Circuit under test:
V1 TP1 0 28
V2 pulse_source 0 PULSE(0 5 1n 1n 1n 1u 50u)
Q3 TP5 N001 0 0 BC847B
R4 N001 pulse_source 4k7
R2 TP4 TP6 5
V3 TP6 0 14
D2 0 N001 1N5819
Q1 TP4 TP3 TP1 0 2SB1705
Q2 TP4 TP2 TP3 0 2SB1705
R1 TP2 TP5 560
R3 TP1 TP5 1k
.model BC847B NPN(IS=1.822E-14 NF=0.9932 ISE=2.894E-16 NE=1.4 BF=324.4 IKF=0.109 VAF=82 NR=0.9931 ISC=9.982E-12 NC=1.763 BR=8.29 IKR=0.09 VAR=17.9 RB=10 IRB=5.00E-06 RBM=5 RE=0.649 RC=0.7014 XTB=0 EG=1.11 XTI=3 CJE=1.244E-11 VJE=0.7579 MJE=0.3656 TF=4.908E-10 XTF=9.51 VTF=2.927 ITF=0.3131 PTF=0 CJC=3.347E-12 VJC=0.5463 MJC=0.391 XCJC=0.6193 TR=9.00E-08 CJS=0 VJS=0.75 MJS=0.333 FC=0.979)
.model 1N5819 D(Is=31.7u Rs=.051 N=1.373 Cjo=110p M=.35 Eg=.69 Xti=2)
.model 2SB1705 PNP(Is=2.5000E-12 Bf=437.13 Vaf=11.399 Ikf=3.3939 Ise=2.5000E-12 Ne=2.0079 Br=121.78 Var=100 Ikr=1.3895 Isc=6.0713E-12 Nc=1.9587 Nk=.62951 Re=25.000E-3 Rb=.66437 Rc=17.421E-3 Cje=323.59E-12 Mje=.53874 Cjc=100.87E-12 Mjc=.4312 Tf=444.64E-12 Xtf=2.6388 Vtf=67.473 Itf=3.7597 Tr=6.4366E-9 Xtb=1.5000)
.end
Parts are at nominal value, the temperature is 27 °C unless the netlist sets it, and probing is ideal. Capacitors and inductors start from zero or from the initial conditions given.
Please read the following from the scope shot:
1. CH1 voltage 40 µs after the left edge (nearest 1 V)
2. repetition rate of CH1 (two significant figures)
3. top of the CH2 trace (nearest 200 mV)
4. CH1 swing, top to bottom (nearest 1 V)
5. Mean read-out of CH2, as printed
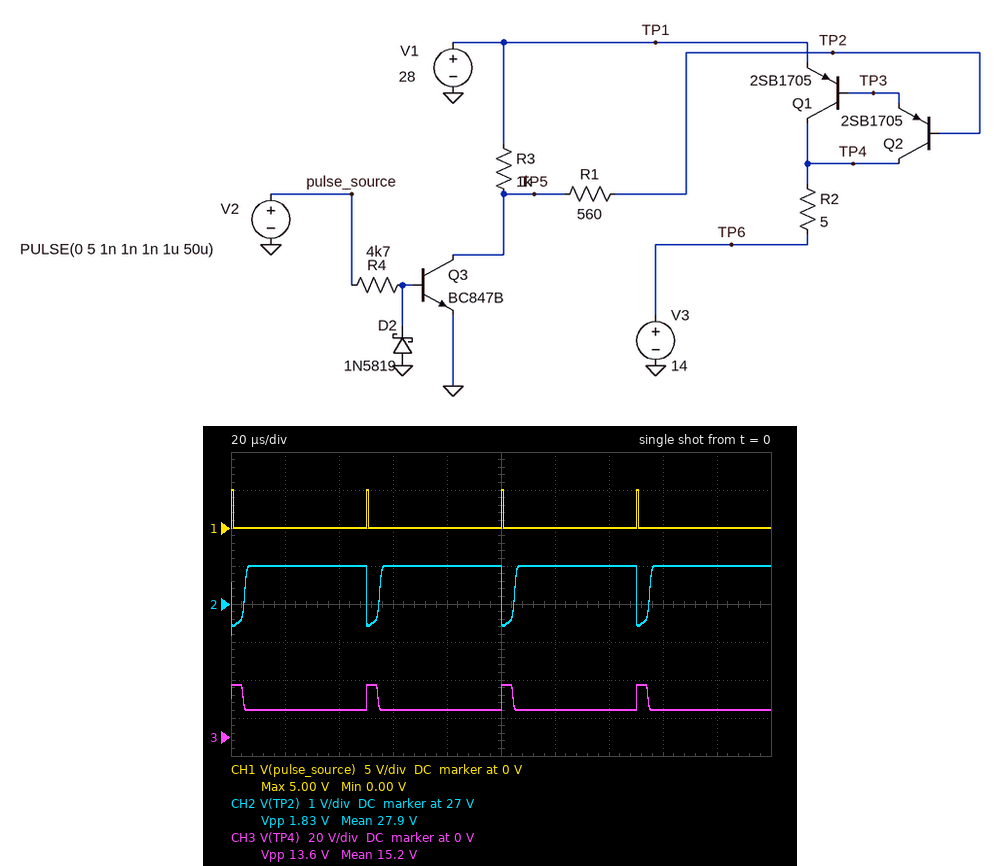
0 V
20 kHz
28.0 V
5 V
27.9 V
